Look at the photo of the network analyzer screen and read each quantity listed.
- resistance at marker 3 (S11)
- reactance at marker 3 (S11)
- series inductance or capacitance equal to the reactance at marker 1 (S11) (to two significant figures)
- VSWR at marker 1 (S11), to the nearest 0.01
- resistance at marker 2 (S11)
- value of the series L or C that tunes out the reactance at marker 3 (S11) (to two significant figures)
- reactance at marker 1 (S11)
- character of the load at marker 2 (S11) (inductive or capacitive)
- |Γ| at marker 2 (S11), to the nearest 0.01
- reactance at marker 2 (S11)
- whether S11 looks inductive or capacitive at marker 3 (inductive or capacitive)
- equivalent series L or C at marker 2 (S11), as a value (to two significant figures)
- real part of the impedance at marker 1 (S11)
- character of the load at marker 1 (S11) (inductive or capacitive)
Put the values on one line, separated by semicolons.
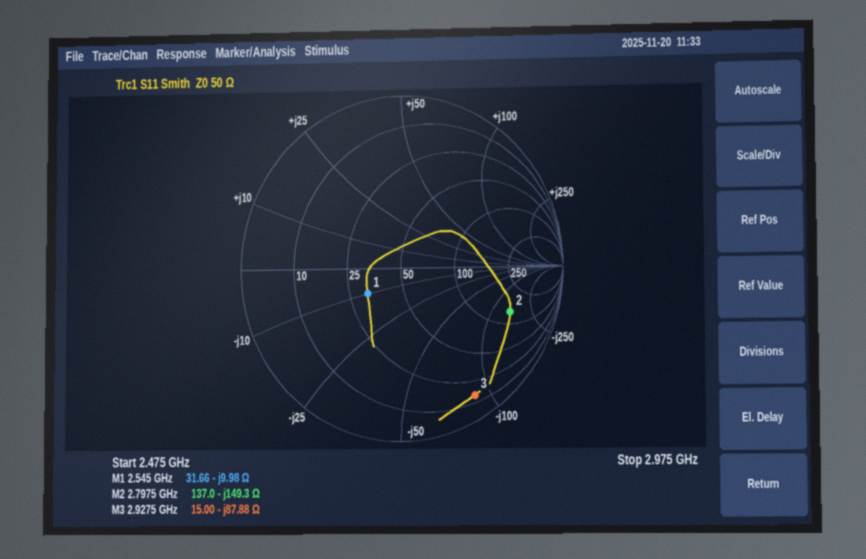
15.00 Ω; -87.88 Ω; 6.3 pF; 1.68; 137.0 Ω; 4.8 nH; -9.98 Ω; capacitive; 0.72; -149.3 Ω; capacitive; 380 fF; 31.66 Ω; capacitive
